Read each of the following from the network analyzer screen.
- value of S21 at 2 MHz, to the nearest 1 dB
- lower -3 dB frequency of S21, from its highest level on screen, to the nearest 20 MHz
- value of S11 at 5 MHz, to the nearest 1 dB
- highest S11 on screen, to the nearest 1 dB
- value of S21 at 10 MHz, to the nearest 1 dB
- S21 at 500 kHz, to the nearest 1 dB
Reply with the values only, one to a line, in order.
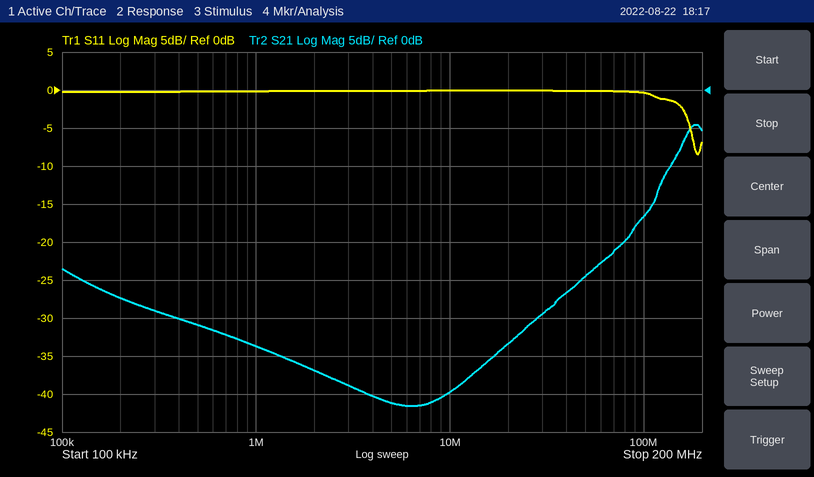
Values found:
-37 dB
160 MHz
0 dB
0 dB
-40 dB
-31 dB
